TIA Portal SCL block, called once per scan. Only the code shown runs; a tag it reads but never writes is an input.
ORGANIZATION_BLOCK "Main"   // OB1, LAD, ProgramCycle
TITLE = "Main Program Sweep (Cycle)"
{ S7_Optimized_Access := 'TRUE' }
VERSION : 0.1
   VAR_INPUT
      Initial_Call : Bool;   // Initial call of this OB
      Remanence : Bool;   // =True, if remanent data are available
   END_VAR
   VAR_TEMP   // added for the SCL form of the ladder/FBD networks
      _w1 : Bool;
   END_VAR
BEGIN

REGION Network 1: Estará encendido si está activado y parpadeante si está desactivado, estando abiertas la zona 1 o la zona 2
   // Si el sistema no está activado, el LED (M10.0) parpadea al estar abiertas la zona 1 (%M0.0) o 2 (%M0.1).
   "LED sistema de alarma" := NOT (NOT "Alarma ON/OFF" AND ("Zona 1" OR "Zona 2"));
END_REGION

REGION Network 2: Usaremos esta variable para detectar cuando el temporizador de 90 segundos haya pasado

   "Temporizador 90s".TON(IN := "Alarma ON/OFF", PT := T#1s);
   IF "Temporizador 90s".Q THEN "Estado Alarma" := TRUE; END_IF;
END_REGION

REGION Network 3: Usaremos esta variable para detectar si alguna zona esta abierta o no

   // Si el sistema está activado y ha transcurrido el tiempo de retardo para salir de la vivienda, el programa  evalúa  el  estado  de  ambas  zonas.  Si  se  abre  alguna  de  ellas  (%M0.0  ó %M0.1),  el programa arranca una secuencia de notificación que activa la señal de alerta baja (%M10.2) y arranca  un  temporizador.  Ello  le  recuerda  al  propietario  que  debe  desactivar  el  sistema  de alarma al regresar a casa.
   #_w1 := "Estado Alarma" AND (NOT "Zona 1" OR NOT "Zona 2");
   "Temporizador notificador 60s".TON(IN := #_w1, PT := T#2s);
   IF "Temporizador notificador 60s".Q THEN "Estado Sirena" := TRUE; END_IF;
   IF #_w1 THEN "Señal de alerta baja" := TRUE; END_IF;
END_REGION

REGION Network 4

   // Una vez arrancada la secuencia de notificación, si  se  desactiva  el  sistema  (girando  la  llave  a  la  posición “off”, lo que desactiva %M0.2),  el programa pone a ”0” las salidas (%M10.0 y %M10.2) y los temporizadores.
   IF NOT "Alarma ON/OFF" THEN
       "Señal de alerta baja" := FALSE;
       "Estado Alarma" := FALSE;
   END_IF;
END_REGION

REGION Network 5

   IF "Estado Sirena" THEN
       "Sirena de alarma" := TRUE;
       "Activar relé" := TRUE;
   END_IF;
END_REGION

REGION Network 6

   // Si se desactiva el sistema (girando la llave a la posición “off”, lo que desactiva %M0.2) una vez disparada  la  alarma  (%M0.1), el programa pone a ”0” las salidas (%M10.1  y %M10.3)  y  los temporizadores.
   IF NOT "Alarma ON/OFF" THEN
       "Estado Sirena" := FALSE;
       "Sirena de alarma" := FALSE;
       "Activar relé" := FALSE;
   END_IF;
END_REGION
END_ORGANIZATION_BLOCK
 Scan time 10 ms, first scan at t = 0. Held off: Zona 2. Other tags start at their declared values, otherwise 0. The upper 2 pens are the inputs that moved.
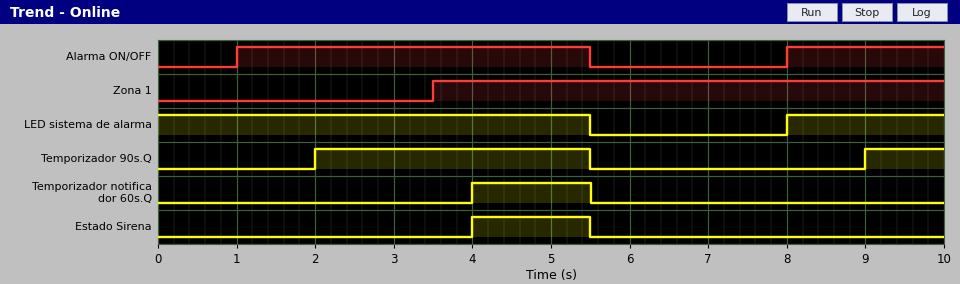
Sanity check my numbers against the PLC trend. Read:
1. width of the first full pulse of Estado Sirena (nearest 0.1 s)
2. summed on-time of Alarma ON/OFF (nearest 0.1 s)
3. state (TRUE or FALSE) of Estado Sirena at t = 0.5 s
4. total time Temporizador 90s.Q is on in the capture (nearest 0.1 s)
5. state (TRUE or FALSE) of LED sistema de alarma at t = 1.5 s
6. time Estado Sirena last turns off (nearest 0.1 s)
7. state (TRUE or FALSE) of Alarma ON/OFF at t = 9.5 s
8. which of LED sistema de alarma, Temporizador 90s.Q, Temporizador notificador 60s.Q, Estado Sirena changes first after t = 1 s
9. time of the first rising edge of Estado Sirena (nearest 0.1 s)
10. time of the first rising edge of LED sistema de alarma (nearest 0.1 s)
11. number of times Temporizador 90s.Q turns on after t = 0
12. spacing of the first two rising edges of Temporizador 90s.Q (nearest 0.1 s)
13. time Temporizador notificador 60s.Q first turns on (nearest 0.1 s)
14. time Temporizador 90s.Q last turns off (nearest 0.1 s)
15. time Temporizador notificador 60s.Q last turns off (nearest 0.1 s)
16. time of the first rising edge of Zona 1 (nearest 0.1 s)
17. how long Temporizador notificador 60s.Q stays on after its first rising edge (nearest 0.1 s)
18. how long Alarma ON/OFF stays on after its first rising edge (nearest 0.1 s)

1.5 s
6.5 s
FALSE
4.5 s
TRUE
5.5 s
TRUE
Temporizador 90s.Q
4.0 s
8.0 s
2
7.0 s
4.0 s
5.5 s
5.5 s
3.5 s
1.5 s
4.5 s
